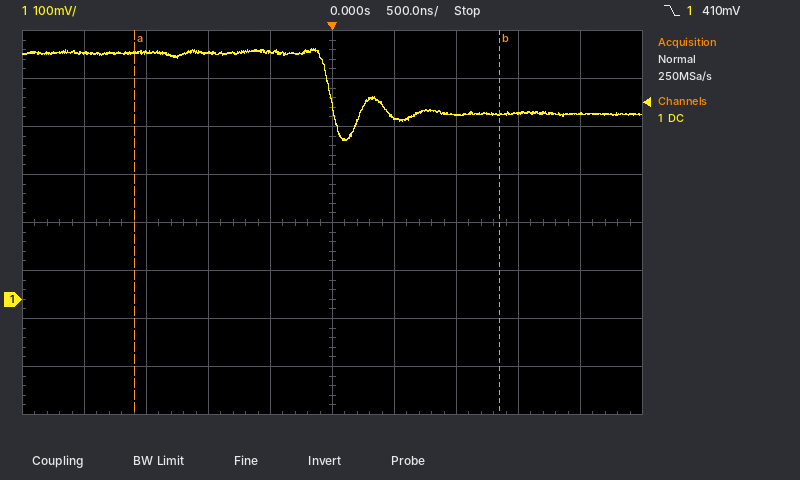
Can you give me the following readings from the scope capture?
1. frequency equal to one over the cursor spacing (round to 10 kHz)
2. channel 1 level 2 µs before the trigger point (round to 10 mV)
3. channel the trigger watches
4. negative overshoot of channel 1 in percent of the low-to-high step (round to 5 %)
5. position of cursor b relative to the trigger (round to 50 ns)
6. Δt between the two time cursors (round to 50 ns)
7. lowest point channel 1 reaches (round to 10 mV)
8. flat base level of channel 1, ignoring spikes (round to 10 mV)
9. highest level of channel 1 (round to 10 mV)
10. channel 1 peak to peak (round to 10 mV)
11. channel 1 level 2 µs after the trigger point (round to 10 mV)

340 kHz
510 mV
channel 1
45 %
+1.35 µs
2.95 µs
330 mV
390 mV
520 mV
190 mV
390 mV
